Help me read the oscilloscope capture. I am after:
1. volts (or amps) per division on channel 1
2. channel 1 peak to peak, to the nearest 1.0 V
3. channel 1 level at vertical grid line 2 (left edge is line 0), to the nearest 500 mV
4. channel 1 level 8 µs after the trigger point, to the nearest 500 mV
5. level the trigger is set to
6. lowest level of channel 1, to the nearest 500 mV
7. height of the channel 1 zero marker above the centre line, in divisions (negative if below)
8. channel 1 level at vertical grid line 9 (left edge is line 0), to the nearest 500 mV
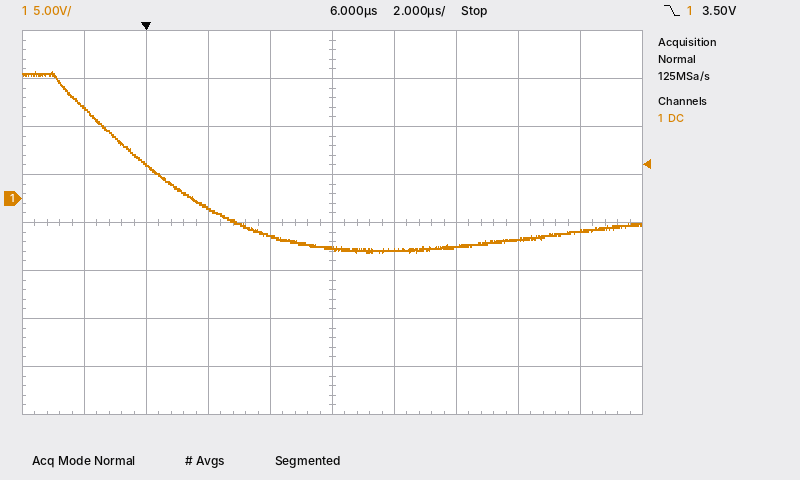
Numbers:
5 V
19.0 V
3.5 V
-5.5 V
3.50 V
-5.5 V
+0.5 div
-3.5 V
